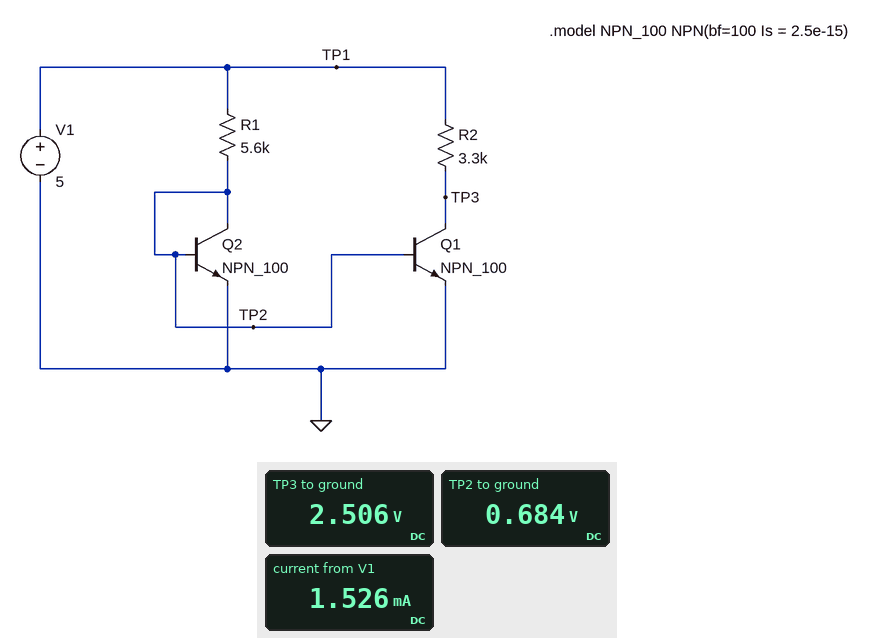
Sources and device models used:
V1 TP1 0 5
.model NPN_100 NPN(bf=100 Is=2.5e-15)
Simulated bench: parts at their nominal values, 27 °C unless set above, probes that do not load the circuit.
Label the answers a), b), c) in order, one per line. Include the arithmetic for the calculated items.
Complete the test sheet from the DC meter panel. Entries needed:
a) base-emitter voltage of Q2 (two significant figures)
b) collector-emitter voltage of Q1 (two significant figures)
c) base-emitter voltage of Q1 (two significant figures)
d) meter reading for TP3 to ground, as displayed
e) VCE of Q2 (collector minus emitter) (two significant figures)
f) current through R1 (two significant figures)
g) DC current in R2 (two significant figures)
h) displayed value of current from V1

a) 684 mV = 680 mV
b) 2.506 V = 2.5 V
c) 684 mV = 680 mV
d) 2.506 V
e) 684 mV = 680 mV
f) (5 V - 684 mV) / 5.6 kΩ = 770 µA
g) (5 V - 2.506 V) / 3.3 kΩ = 760 µA
h) 1.526 mA
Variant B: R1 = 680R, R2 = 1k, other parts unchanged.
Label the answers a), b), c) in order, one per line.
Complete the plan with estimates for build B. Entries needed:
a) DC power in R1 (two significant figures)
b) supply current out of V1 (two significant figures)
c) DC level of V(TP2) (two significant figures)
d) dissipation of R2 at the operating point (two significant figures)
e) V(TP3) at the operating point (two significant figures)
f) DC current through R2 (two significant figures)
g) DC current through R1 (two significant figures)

a) 27 mW
b) 11 mA
c) 740 mV
d) 24 mW
e) 68 mV
f) 4.9 mA
g) 6.3 mA
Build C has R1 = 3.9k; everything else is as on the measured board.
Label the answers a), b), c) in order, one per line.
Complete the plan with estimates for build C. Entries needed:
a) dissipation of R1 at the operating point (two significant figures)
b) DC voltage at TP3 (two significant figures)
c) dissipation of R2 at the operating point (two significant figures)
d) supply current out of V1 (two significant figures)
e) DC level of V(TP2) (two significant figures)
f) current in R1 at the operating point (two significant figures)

a) 4.8 mW
b) 1.4 V
c) 3.9 mW
d) 2.2 mA
e) 690 mV
f) 1.1 mA
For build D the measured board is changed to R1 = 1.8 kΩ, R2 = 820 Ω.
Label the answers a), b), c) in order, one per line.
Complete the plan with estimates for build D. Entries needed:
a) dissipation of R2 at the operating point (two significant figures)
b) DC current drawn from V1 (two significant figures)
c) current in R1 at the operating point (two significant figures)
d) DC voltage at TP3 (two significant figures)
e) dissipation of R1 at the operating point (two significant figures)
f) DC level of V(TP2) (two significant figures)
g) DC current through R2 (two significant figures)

a) 4.5 mW
b) 4.7 mA
c) 2.4 mA
d) 3.1 V
e) 10 mW
f) 710 mV
g) 2.3 mA
